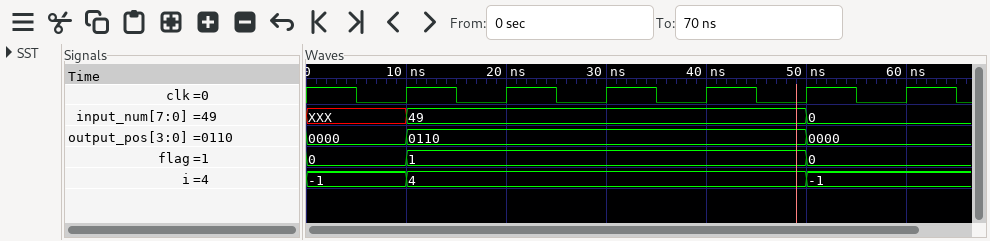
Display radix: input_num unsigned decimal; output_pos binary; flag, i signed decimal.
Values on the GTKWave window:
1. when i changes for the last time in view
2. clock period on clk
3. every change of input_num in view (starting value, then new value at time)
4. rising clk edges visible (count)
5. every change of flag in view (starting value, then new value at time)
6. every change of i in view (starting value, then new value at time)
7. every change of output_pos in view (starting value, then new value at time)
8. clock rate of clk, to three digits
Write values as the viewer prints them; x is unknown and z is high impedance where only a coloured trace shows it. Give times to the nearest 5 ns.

50 ns
10 ns
XXX, 49 at 10 ns, 0 at 50 ns
6
0, 1 at 10 ns, 0 at 50 ns
-1, 4 at 10 ns, -1 at 50 ns
0000, 0110 at 10 ns, 0000 at 50 ns
100 MHz
